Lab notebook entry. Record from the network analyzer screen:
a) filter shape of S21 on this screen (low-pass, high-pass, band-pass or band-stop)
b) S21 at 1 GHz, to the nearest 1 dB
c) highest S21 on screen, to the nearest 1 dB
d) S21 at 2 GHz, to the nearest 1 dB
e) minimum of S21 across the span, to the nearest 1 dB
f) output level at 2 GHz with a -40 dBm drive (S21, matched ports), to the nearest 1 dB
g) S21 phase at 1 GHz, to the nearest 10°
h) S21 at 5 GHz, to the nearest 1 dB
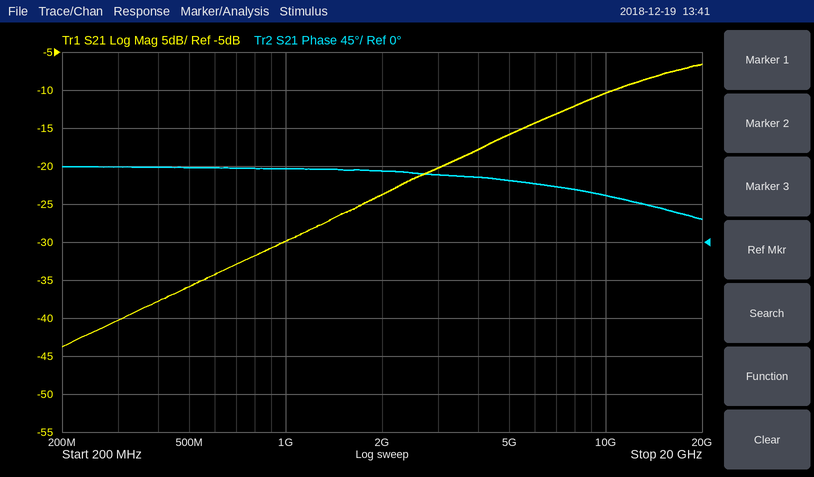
high-pass
-30 dB
-7 dB
-24 dB
-44 dB
-64 dBm
90°
-16 dB
